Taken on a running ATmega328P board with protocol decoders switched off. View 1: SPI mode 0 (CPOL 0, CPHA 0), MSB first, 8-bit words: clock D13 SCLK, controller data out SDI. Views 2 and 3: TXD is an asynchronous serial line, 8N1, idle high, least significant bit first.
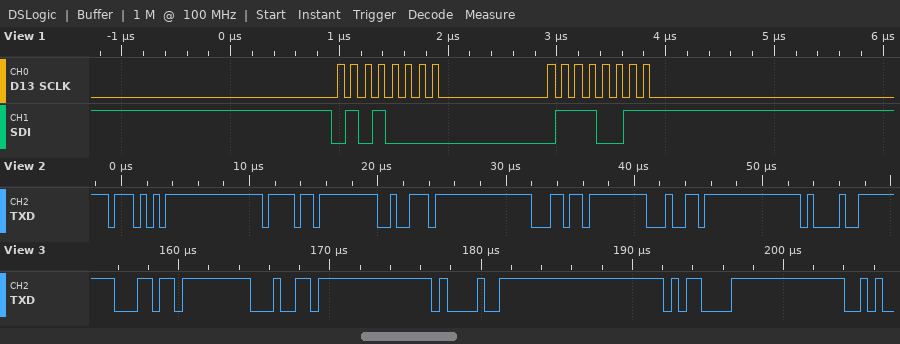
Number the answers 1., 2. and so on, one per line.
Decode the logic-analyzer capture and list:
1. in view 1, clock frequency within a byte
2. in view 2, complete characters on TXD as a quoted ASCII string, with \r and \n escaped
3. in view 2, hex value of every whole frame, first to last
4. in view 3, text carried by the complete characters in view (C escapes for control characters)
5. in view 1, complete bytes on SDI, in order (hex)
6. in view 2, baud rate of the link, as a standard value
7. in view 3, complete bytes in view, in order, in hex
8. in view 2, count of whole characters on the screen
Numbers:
1. 8 MHz
2. "World!"
3. 57 6F 72 6C 64 21
4. "ld!\r"
5. 50 73
6. 2000000 baud
7. 6C 64 21 0D
8. 6
